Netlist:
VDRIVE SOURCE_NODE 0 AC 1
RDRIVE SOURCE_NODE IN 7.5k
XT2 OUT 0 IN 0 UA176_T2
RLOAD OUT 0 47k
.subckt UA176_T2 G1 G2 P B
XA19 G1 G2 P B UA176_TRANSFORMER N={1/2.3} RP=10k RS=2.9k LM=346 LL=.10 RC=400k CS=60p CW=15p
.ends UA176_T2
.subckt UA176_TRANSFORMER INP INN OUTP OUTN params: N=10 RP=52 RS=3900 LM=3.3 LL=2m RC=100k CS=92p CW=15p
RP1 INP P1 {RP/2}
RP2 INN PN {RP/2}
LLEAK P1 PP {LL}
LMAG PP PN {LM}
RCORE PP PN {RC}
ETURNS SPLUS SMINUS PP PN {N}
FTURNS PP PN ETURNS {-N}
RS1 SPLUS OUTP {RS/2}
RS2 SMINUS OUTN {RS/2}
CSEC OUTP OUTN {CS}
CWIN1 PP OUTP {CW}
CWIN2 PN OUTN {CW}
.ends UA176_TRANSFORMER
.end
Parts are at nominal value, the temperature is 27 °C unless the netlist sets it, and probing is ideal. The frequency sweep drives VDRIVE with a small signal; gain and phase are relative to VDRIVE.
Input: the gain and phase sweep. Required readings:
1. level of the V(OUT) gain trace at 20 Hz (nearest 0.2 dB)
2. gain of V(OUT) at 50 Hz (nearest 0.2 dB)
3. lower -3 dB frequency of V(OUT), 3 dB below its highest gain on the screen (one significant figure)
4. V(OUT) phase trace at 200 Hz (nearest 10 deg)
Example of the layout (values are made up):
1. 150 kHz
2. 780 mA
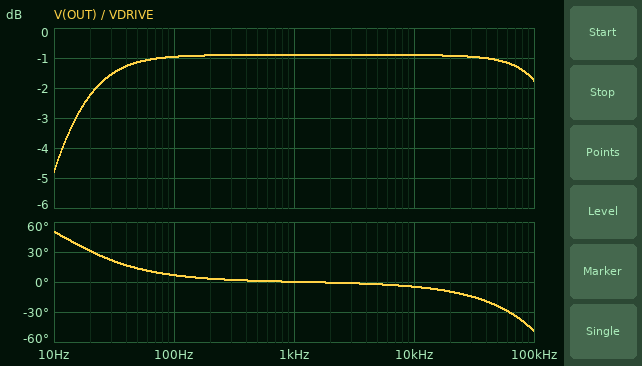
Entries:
1. -2.2 dB
2. -1.2 dB
3. 10 Hz
4. 0 deg
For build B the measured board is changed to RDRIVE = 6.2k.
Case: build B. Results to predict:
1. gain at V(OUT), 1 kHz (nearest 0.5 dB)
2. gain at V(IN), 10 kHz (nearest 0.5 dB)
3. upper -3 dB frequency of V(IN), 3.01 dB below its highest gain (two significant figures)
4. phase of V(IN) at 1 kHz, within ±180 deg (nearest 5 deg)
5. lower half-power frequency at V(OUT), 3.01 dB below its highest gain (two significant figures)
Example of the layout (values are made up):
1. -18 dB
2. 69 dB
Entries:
1. -0.5 dB
2. -3.5 dB
3. 450 kHz
4. 0 deg
5. 11 Hz
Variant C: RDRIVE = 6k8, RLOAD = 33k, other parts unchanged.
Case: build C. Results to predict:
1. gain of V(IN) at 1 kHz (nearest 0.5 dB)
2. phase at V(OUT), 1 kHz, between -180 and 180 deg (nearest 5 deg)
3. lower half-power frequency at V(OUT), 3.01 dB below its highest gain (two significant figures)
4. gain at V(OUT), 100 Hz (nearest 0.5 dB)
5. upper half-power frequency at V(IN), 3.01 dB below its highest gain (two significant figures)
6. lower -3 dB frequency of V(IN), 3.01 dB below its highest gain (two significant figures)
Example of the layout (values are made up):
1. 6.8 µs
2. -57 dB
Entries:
1. -4.5 dB
2. 0 deg
3. 10 Hz
4. -2.5 dB
5. 410 kHz
6. 31 Hz
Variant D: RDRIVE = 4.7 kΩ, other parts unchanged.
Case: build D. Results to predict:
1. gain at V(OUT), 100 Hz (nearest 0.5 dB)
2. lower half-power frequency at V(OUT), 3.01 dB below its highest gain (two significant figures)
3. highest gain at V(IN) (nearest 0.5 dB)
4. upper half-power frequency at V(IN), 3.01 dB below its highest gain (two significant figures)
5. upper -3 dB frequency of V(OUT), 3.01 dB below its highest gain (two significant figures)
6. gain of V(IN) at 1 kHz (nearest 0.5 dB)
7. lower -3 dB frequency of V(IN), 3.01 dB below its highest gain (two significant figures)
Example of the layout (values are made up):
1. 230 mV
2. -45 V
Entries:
1. 0.5 dB
2. 10 Hz
3. -1.5 dB
4. 550 kHz
5. 160 kHz
6. -3.0 dB
7. 12 Hz
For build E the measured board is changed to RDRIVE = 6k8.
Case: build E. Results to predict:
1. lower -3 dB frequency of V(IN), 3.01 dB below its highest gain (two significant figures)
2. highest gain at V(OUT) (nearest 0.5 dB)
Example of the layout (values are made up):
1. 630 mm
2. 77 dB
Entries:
1. 18 Hz
2. -0.5 dB
